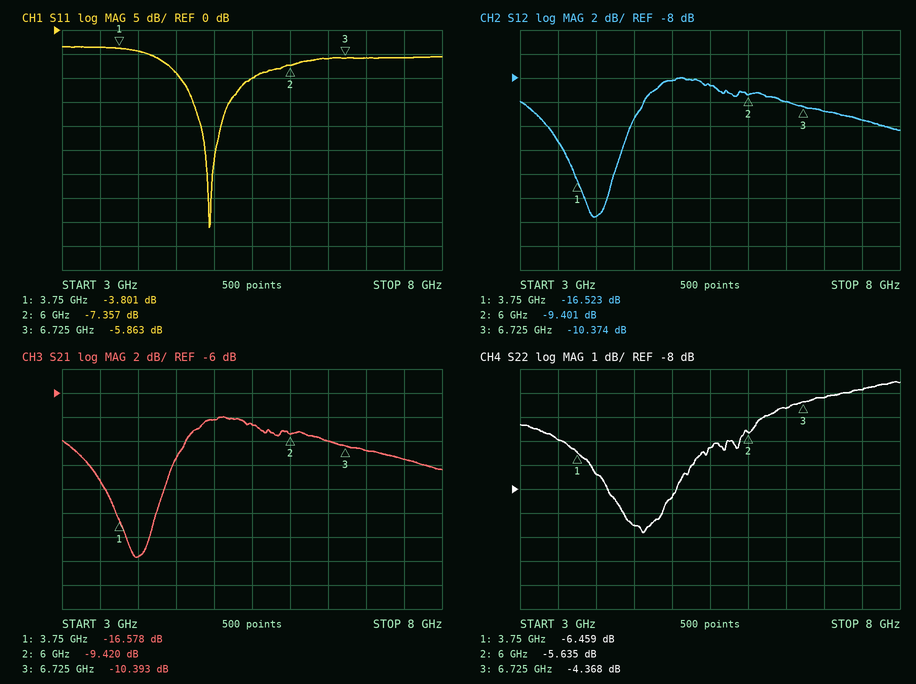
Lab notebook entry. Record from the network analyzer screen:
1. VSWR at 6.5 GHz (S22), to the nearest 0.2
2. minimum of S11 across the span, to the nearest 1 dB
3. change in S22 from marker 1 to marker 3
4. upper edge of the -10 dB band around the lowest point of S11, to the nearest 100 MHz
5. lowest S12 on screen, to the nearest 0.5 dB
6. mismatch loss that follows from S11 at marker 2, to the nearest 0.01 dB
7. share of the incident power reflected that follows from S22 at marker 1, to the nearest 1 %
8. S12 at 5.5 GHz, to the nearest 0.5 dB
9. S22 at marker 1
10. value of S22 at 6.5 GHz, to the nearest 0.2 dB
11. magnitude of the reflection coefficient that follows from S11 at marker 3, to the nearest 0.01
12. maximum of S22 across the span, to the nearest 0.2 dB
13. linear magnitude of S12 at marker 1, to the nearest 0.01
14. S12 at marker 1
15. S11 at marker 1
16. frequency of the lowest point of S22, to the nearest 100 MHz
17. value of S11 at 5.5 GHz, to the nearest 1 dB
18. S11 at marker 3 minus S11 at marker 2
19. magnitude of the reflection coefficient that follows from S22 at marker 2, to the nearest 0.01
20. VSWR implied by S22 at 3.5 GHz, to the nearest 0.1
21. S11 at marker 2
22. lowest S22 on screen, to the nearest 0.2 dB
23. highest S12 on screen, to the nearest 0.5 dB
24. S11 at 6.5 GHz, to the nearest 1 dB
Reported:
3.8
-41 dB
2.091 dB
5.5 GHz
-19.5 dB
0.88 dB
23 %
-8.5 dB
-6.459 dB
-4.6 dB
0.51
-3.6 dB
0.15
-16.523 dB
-3.801 dB
4.6 GHz
-10 dB
1.494 dB
0.52
3.0
-7.357 dB
-9.8 dB
-8.0 dB
-6 dB
